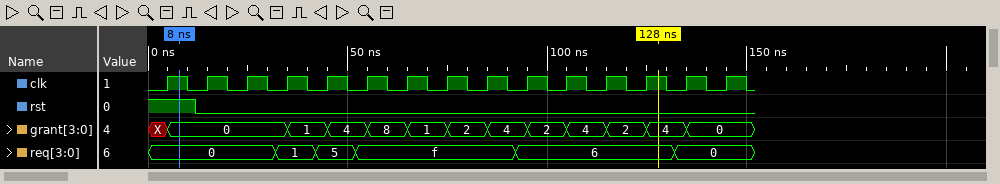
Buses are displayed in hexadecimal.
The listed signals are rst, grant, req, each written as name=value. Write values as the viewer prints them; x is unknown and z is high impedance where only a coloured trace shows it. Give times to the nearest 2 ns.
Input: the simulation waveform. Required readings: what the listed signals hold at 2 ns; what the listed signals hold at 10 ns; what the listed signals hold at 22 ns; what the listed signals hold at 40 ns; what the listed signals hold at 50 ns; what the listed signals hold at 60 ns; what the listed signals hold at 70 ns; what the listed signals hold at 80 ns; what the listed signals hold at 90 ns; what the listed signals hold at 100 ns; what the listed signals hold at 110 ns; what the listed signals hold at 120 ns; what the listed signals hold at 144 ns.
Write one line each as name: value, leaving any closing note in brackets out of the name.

what the listed signals hold at 2 ns: rst=1, grant=X, req=0
what the listed signals hold at 10 ns: rst=1, grant=0, req=0
what the listed signals hold at 22 ns: rst=0, grant=0, req=0
what the listed signals hold at 40 ns: rst=0, grant=1, req=1
what the listed signals hold at 50 ns: rst=0, grant=4, req=5
what the listed signals hold at 60 ns: rst=0, grant=8, req=f
what the listed signals hold at 70 ns: rst=0, grant=1, req=f
what the listed signals hold at 80 ns: rst=0, grant=2, req=f
what the listed signals hold at 90 ns: rst=0, grant=4, req=f
what the listed signals hold at 100 ns: rst=0, grant=2, req=6
what the listed signals hold at 110 ns: rst=0, grant=4, req=6
what the listed signals hold at 120 ns: rst=0, grant=2, req=6
what the listed signals hold at 144 ns: rst=0, grant=0, req=0
